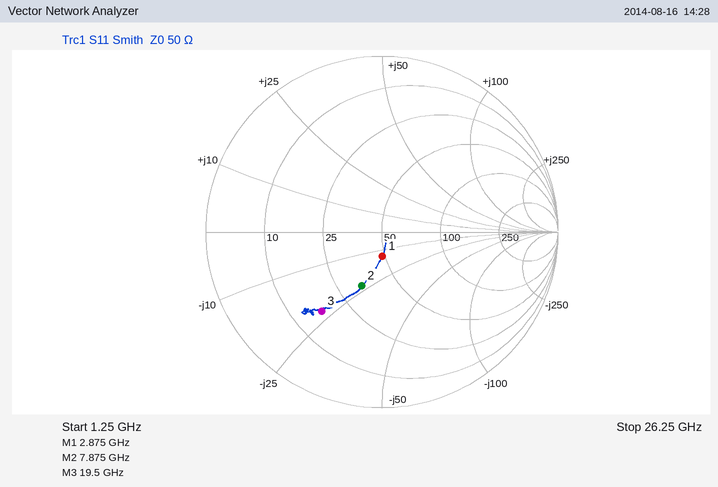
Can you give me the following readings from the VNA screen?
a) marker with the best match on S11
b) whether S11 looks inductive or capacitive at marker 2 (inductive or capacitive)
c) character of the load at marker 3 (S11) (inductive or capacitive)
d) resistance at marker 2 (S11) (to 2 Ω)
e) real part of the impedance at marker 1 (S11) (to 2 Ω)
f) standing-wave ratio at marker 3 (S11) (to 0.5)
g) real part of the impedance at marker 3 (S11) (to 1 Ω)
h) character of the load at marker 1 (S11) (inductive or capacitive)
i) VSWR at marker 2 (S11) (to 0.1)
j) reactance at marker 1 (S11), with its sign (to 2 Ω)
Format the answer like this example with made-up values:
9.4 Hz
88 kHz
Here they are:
marker 1
capacitive
capacitive
34 Ω
48 Ω
3.5
17 Ω
capacitive
2.0
-14 Ω
